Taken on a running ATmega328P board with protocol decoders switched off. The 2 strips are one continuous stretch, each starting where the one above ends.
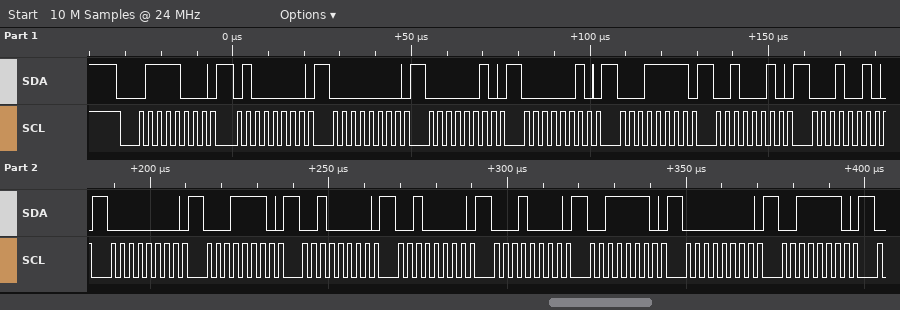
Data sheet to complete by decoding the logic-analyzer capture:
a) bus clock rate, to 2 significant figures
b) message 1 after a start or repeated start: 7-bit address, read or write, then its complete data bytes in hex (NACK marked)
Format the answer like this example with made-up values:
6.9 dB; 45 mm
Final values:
400 kHz; 0x3C write: 40 00 02 02 1F 22 12 00 1E 20 20 10 3E 00 3E
